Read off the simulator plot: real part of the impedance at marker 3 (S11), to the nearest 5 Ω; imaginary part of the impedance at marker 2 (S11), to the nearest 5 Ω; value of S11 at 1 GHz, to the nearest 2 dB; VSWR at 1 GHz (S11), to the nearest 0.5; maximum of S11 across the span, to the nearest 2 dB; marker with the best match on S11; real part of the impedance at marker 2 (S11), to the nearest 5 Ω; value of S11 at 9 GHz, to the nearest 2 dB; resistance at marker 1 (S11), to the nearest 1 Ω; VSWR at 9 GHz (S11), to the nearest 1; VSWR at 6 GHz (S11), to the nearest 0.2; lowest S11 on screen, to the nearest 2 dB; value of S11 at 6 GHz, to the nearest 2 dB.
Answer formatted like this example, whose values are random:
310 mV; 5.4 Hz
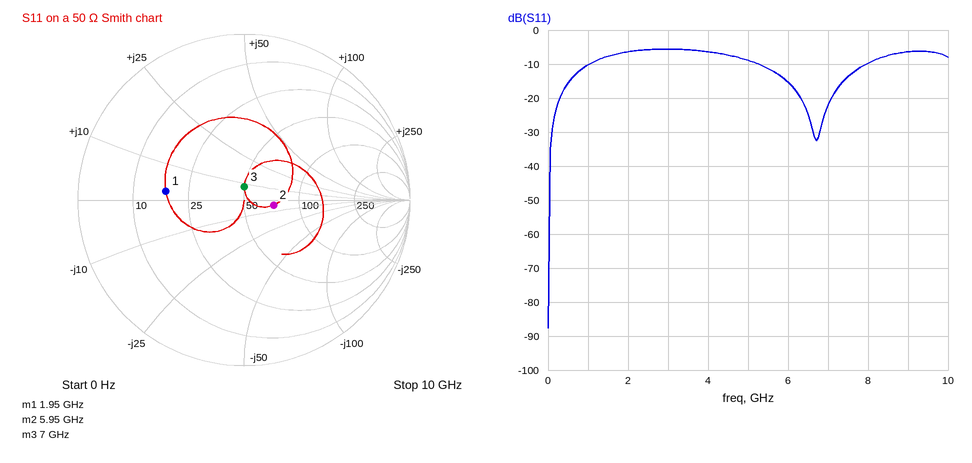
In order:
50 Ω; -5 Ω; -10 dB; 2.0; -6 dB; marker 3; 70 Ω; -6 dB; 18 Ω; 3; 1.4; -88 dB; -16 dB
